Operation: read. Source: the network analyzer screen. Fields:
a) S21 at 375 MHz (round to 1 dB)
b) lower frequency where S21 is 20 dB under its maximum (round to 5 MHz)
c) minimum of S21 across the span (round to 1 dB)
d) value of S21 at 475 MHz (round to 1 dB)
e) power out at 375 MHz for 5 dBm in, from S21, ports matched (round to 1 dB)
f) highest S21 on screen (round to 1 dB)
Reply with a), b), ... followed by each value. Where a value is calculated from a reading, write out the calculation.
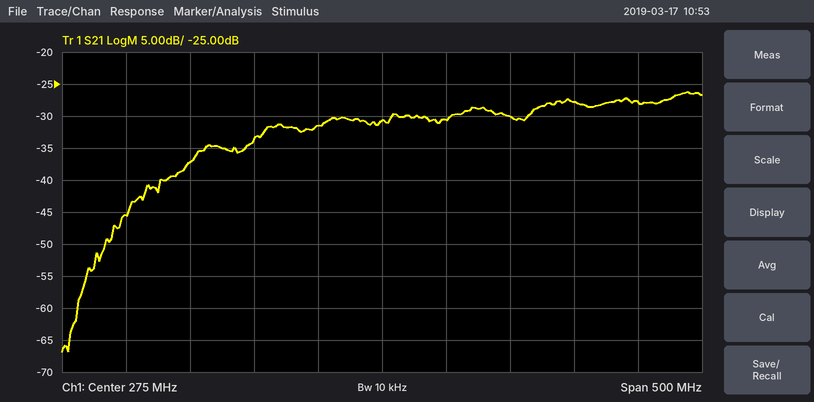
a) -30 dB
b) 70 MHz
c) -67 dB
d) -28 dB
e) 5 dBm + (-30 dB) = -25 dBm
f) -26 dB
